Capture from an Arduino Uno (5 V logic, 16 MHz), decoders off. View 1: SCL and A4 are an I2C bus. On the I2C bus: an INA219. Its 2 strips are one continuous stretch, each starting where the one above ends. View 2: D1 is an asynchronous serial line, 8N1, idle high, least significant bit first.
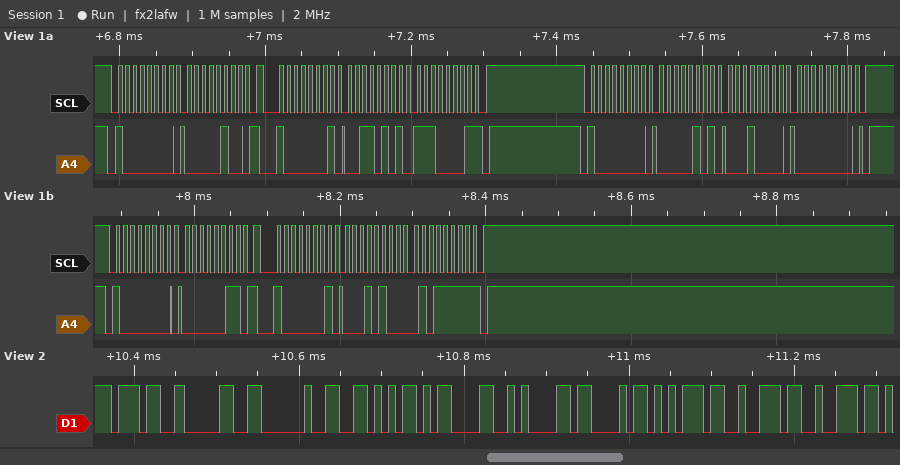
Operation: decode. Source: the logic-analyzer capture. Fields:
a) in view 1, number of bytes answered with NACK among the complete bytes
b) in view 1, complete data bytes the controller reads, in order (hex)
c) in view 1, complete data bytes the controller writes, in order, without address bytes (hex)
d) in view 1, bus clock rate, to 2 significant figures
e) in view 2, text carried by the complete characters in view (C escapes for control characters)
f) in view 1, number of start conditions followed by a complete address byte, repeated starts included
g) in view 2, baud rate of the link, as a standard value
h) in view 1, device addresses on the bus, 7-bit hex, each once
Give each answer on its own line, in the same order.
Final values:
2
35 E1 14 5F
04 05 10 00 03
100 kHz
"70 V\r\nCurr"
5
115200 baud
0x40
